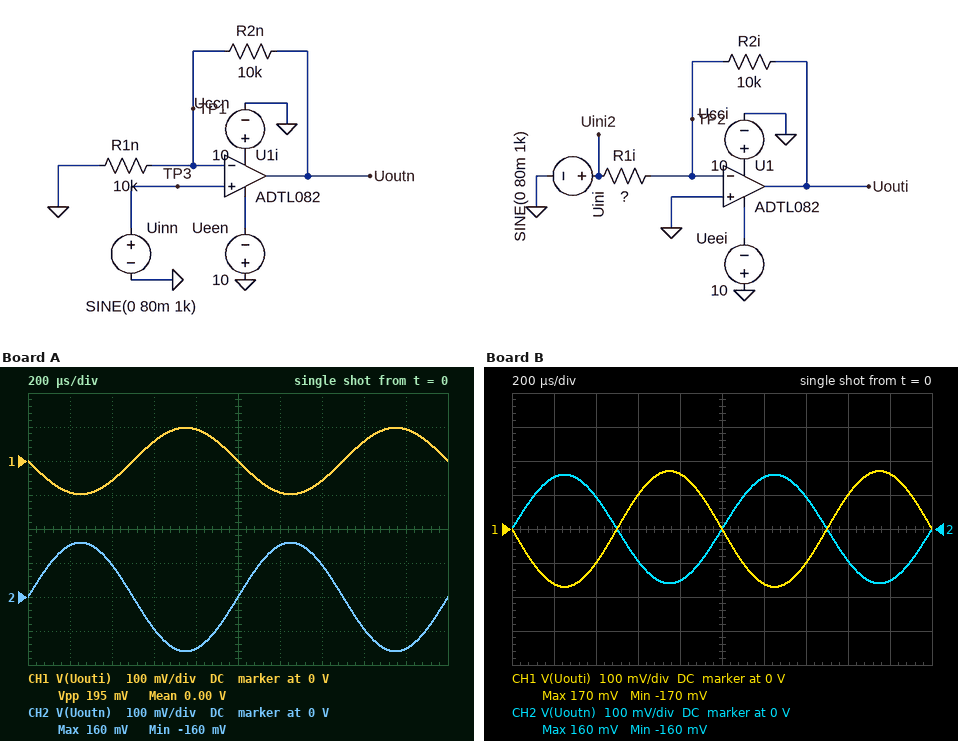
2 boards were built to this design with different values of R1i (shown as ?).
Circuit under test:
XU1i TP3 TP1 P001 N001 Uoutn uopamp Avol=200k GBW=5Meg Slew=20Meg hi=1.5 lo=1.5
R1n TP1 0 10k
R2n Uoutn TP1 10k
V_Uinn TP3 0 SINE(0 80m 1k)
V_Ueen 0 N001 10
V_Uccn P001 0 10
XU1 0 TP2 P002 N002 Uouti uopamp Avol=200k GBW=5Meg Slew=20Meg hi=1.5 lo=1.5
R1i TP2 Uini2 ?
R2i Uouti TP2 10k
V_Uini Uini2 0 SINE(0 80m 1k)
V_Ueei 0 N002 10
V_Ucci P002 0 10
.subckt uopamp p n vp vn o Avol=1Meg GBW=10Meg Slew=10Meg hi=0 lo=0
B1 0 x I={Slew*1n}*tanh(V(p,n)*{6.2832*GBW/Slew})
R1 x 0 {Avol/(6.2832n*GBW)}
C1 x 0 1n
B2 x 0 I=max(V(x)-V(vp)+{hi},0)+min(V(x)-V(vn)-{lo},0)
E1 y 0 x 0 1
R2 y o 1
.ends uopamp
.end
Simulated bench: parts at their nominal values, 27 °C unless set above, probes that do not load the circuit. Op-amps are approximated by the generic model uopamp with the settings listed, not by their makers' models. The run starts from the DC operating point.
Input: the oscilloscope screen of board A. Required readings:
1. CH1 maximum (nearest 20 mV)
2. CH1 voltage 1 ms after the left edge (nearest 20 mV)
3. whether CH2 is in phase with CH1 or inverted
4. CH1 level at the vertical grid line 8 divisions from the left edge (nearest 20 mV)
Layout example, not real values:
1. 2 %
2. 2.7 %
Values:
1. 100 mV
2. 0 V
3. inverted
4. 60 mV
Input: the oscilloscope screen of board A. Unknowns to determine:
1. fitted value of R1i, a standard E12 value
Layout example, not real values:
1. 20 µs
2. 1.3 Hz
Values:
1. 8.2 kΩ
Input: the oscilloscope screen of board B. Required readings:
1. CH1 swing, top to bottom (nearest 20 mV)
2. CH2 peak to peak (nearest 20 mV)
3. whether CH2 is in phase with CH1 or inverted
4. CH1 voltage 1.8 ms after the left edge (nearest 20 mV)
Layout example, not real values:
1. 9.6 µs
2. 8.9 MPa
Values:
1. 340 mV
2. 320 mV
3. inverted
4. 160 mV
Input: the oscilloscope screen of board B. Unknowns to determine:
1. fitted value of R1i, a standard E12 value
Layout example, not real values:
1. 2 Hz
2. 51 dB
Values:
1. 4.7 kΩ
